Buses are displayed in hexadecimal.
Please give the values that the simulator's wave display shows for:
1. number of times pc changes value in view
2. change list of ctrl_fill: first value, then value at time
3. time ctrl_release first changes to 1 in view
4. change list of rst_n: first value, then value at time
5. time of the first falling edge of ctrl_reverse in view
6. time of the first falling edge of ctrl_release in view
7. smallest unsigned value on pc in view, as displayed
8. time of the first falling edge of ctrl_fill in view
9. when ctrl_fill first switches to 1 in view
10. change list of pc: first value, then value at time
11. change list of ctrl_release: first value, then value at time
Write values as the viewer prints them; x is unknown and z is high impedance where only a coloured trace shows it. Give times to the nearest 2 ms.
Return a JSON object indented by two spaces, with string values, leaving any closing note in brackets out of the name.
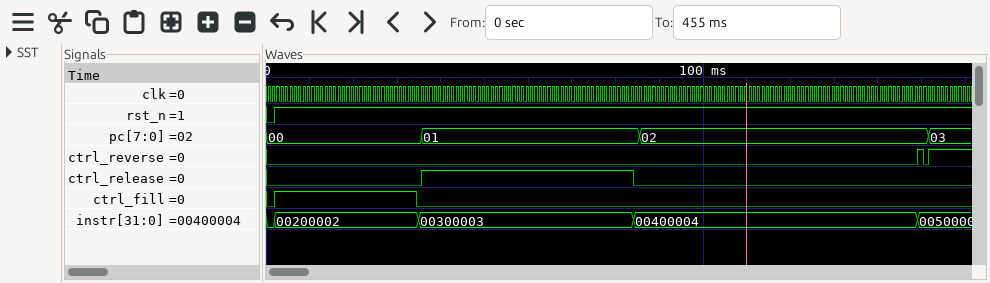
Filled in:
{
  "number of times pc changes value in view": "3",
  "change list of ctrl_fill: first value, then value at time": "0, 1 at 2 ms, 0 at 34 ms",
  "time ctrl_release first changes to 1 in view": "36 ms",
  "change list of rst_n: first value, then value at time": "0, 1 at 2 ms",
  "time of the first falling edge of ctrl_reverse in view": "150 ms",
  "time of the first falling edge of ctrl_release in view": "84 ms",
  "smallest unsigned value on pc in view, as displayed": "00",
  "time of the first falling edge of ctrl_fill in view": "34 ms",
  "when ctrl_fill first switches to 1 in view": "2 ms",
  "change list of pc: first value, then value at time": "00, 01 at 36 ms, 02 at 86 ms, 03 at 152 ms",
  "change list of ctrl_release: first value, then value at time": "0, 1 at 36 ms, 0 at 84 ms"
}
